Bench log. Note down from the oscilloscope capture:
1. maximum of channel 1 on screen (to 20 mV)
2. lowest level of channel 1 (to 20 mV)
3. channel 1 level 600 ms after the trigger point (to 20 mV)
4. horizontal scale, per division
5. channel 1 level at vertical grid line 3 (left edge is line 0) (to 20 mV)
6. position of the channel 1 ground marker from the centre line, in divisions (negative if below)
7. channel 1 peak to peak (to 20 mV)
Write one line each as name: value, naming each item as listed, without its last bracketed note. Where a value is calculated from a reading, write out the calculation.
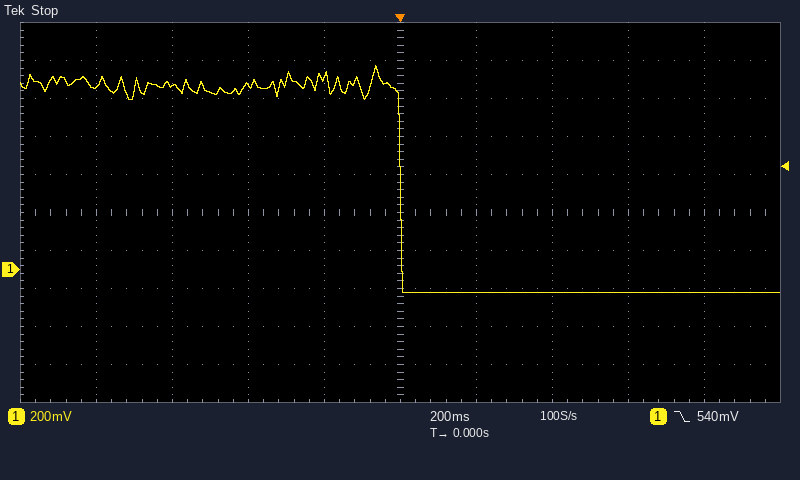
maximum of channel 1 on screen: 1.08 V
lowest level of channel 1: -120 mV
channel 1 level 600 ms after the trigger point: -120 mV
horizontal scale, per division: 200 ms
channel 1 level at vertical grid line 3 (left edge is line 0): 960 mV
position of the channel 1 ground marker from the centre line, in divisions: -1.5 div
channel 1 peak to peak: 1.08 V − (-120 mV) = 1.20 V
